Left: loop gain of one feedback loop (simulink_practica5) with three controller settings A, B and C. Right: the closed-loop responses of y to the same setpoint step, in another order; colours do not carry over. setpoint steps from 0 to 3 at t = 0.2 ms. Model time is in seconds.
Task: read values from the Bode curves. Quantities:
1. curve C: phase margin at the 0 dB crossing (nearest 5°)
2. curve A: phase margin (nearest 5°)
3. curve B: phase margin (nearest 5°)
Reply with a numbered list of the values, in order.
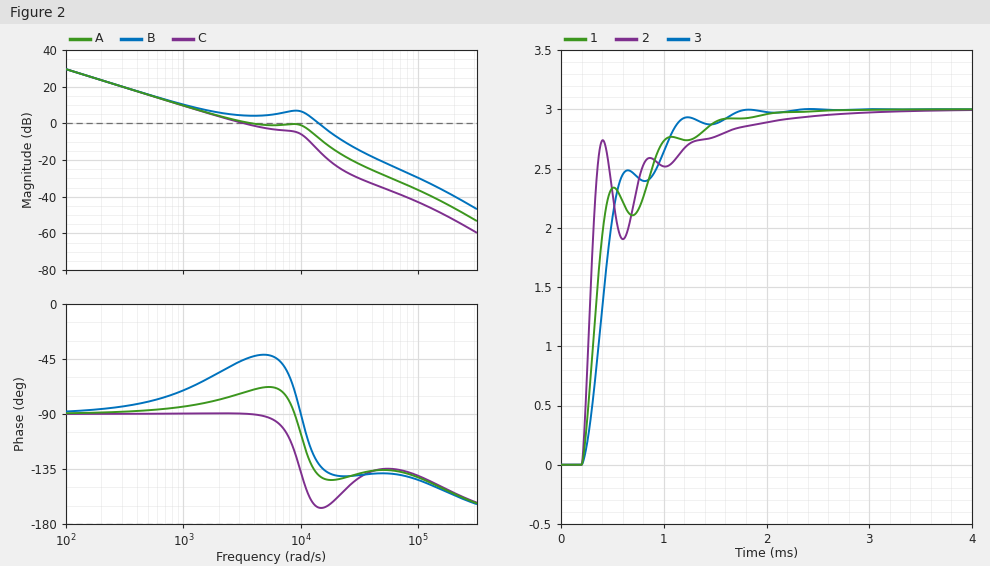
1. 90°
2. 110°
3. 50°
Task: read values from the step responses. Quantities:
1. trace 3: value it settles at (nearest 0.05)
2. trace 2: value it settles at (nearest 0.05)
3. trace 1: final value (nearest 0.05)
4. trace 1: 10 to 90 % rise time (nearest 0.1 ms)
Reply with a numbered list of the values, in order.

1. 3.00
2. 3.00
3. 3.00
4. 0.7 ms
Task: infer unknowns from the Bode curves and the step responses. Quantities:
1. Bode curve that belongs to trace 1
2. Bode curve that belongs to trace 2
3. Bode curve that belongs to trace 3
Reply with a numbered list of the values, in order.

1. A
2. B
3. C
